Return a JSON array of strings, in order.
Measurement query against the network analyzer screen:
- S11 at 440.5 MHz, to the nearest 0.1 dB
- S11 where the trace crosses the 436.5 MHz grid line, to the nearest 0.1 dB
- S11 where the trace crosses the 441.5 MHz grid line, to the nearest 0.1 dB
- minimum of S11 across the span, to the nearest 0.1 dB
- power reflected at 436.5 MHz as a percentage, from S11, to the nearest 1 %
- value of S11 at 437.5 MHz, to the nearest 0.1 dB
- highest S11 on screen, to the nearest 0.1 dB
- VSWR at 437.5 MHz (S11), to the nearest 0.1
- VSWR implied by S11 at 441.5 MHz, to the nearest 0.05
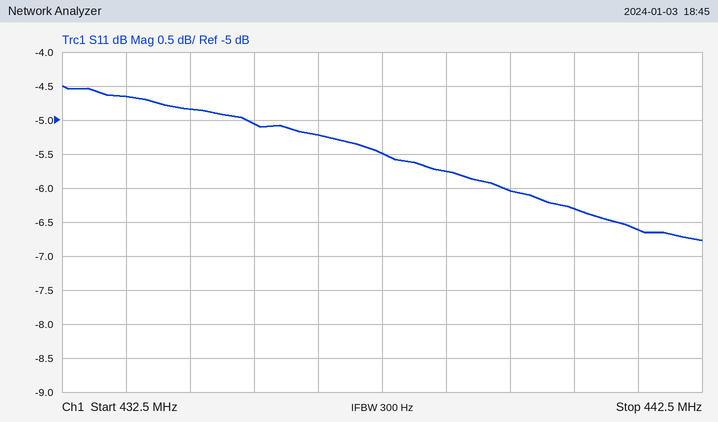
["-6.3 dB", "-5.2 dB", "-6.6 dB", "-6.8 dB", "30 %", "-5.5 dB", "-4.5 dB", "3.3", "2.75"]
